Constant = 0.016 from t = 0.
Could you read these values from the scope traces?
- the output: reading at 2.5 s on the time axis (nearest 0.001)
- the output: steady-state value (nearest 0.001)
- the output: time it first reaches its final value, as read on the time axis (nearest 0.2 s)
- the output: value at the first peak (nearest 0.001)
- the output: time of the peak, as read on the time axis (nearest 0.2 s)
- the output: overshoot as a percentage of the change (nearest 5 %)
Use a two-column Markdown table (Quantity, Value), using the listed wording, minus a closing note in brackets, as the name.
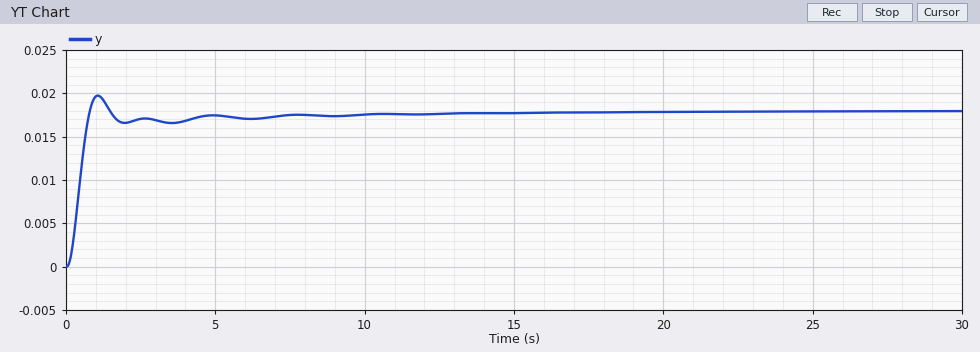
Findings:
| Quantity | Value |
|---|---|
| the output: reading at 2.5 s on the time axis | 0.017 |
| the output: steady-state value | 0.018 |
| the output: time it first reaches its final value, as read on the time axis | 0.8 s |
| the output: value at the first peak | 0.020 |
| the output: time of the peak, as read on the time axis | 1.0 s |
| the output: overshoot as a percentage of the change | 10 % |
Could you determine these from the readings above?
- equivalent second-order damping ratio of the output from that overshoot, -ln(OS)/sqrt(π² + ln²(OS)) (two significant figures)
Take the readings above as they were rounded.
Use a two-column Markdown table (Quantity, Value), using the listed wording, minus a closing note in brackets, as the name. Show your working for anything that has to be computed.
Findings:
| Quantity | Value |
|---|---|
| equivalent second-order damping ratio of the output from that overshoot, -ln(OS)/sqrt(π² + ln²(OS)) | ln(0.1) = -2.303; 2.303 / sqrt(9.870 + 5.302) = 0.59 |
